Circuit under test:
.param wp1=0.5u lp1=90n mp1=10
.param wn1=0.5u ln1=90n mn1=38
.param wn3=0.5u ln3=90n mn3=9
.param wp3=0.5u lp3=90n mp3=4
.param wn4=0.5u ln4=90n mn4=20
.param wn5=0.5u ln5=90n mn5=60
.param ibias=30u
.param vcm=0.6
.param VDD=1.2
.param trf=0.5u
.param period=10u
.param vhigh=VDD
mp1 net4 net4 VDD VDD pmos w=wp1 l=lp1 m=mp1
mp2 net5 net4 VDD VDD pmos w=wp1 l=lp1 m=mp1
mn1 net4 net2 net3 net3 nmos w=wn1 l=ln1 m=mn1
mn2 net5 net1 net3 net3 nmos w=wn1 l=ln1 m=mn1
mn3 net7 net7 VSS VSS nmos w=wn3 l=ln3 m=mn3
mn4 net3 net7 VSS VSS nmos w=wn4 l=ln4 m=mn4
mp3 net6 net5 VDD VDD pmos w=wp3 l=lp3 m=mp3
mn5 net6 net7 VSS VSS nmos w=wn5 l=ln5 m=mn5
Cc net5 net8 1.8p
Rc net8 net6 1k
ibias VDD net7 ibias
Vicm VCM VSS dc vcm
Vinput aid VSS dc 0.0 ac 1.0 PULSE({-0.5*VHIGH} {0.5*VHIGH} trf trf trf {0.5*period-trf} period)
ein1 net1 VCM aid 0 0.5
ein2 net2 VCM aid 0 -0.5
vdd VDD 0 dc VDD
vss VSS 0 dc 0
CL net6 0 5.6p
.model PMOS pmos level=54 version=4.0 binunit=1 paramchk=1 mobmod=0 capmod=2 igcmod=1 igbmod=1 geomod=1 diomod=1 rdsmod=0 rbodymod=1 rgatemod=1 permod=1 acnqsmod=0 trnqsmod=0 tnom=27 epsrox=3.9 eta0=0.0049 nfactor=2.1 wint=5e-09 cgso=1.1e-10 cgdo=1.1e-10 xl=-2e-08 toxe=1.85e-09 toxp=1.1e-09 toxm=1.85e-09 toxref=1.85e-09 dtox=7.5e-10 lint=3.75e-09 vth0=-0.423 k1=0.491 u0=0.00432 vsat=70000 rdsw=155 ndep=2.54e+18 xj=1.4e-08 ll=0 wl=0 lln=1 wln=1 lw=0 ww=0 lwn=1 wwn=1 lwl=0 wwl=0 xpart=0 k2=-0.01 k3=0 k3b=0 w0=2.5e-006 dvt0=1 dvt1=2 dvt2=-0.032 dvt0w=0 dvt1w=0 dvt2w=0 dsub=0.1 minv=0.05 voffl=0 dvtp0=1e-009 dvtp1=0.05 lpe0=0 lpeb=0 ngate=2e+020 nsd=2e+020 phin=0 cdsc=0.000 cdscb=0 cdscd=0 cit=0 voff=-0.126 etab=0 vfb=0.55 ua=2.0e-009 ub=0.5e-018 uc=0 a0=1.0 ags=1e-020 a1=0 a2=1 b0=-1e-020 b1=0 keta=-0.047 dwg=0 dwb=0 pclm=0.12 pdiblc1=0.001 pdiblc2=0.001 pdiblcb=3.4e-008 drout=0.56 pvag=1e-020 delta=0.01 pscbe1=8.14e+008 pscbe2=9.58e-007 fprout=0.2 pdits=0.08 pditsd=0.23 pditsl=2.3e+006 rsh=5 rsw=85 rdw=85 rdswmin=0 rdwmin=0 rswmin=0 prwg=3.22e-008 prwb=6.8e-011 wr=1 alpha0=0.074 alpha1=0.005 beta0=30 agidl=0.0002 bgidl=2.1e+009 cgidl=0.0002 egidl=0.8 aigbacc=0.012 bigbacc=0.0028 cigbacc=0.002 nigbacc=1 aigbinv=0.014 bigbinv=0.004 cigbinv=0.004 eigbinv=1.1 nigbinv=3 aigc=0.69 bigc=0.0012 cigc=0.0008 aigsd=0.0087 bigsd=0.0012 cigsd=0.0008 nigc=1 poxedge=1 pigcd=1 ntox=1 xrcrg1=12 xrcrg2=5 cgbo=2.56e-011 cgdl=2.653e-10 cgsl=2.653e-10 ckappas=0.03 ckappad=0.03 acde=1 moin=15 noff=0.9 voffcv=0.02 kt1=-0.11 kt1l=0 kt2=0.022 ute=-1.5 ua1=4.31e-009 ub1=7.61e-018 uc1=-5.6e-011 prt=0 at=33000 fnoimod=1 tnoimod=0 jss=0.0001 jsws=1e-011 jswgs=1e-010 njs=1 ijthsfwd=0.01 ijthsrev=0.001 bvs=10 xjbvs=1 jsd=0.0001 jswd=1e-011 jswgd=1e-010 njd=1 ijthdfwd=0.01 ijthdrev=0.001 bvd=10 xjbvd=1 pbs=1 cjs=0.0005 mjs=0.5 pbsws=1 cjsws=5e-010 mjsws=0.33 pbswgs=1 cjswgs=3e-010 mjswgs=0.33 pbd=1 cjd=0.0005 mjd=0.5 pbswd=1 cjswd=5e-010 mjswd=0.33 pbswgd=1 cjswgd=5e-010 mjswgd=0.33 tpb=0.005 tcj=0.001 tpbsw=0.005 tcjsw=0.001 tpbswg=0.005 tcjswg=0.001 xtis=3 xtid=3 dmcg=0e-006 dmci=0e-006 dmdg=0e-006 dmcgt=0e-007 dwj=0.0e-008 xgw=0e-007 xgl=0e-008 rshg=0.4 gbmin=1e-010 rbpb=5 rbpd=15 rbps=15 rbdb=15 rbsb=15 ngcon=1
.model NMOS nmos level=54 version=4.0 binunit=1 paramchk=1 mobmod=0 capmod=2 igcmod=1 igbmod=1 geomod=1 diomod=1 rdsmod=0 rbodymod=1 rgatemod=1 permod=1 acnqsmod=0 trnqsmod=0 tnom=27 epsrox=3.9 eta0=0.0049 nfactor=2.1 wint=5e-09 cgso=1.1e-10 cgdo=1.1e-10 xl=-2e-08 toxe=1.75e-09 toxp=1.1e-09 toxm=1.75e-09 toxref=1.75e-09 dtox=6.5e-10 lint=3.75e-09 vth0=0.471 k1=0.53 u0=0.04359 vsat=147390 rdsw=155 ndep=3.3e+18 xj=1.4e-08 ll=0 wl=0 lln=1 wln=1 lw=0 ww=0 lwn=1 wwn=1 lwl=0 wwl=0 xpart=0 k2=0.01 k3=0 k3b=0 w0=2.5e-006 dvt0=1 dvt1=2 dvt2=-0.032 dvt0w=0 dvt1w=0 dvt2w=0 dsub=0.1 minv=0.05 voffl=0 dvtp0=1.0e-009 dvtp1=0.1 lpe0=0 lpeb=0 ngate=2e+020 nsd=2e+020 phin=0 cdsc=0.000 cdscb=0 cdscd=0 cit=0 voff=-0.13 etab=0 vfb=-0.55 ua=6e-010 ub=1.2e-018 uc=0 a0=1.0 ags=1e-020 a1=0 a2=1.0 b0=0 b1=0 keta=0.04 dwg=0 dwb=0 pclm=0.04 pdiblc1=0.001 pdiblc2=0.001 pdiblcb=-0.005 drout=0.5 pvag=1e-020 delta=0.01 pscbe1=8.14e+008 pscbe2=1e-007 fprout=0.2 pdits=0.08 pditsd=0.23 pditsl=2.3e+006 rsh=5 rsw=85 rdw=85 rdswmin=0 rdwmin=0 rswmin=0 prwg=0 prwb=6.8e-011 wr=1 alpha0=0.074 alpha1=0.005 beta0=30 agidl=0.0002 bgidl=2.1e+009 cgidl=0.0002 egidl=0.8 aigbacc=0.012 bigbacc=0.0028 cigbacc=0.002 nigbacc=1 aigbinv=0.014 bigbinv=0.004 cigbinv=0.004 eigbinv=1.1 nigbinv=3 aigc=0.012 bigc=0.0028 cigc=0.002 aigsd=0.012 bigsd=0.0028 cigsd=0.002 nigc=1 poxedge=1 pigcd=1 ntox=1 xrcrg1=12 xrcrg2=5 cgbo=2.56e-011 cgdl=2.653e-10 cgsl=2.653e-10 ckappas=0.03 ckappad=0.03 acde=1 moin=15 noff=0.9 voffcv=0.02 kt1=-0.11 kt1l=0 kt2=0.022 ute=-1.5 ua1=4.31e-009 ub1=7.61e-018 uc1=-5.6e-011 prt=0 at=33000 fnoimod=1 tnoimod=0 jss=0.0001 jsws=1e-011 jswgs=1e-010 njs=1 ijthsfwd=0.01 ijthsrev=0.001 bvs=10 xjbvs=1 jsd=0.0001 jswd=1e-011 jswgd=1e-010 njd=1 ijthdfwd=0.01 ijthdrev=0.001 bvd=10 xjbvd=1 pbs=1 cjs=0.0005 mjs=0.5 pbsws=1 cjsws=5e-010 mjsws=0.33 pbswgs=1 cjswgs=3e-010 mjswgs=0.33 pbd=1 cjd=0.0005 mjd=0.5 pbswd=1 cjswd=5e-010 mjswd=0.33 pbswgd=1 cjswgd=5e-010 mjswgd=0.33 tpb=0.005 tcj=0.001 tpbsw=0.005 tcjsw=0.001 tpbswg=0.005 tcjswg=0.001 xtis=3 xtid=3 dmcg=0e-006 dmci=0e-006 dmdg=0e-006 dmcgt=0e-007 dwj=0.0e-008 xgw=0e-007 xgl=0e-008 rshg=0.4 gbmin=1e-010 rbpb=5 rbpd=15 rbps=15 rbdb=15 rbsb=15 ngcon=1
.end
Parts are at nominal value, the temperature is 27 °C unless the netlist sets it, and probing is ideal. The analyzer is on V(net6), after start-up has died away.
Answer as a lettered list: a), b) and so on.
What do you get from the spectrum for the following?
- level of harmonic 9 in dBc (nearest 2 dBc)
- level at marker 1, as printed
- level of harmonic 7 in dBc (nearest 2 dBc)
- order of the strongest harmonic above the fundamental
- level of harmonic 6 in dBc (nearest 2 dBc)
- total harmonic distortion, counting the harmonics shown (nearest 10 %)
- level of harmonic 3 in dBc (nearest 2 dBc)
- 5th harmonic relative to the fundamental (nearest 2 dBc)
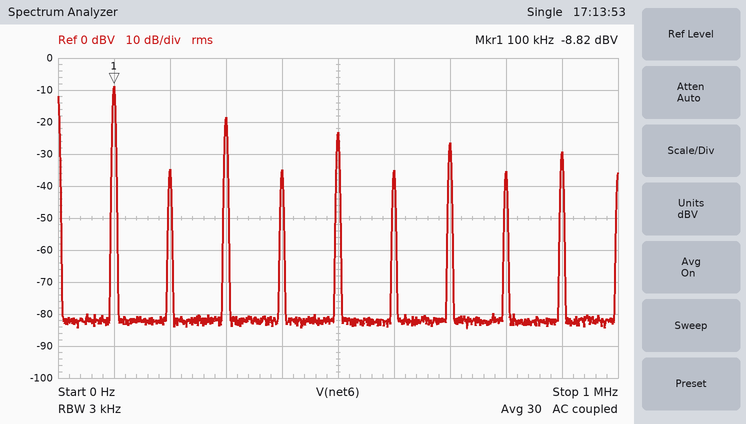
a) -20 dBc
b) -8.82 dBV
c) -18 dBc
d) 3
e) -26 dBc
f) 40 %
g) -10 dBc
h) -14 dBc
